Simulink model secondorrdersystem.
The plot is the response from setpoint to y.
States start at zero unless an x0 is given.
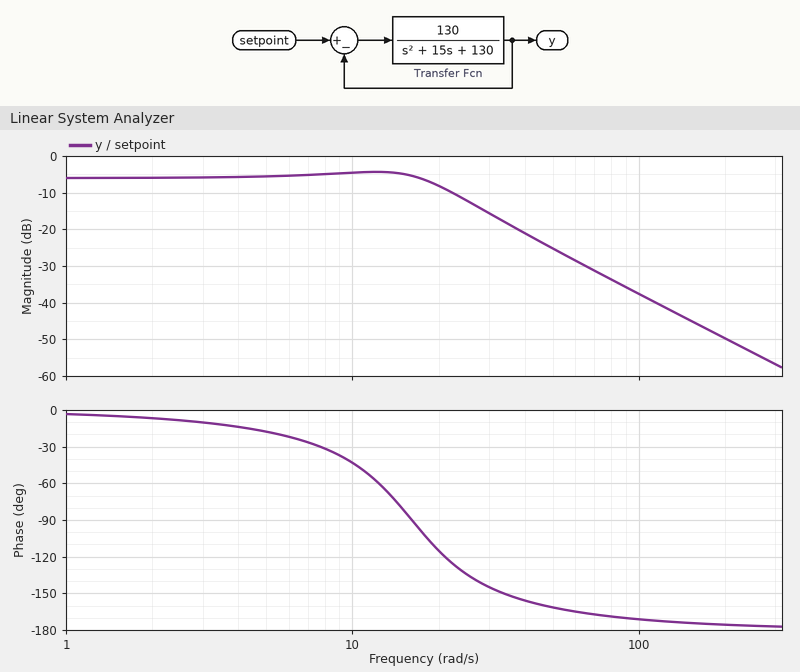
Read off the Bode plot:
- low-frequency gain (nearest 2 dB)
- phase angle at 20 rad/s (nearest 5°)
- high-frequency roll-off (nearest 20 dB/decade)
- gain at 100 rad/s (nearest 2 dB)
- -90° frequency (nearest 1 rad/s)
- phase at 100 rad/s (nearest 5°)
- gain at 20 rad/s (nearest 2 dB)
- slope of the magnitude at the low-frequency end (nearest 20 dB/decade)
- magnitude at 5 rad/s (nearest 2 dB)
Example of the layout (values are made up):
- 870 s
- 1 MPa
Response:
- -6 dB
- -115°
- -40 dB/decade
- -38 dB
- 16 rad/s
- -170°
- -8 dB
- 0 dB/decade
- -6 dB
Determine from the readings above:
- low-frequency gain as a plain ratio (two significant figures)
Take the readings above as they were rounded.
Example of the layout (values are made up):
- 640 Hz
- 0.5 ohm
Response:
- 0.50
